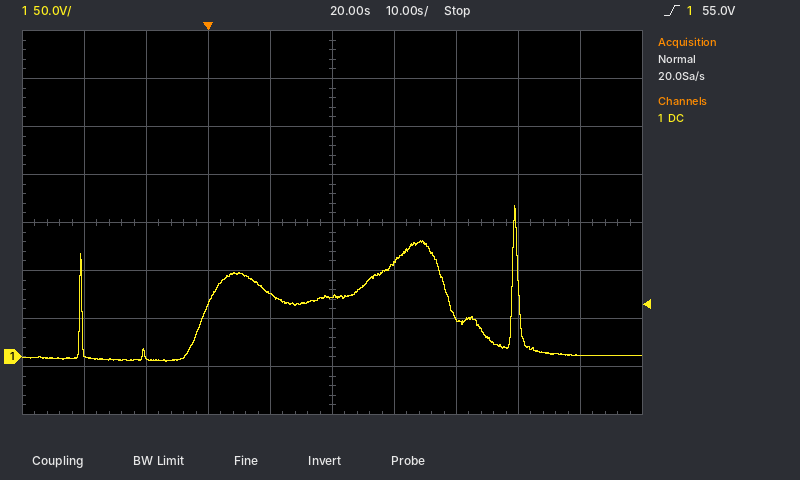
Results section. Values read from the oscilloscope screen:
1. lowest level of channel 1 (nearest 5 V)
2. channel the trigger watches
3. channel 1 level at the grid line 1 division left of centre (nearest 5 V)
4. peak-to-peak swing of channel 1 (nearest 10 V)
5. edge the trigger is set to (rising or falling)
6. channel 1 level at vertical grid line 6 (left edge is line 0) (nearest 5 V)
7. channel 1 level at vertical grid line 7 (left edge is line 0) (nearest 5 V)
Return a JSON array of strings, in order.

["-5 V", "channel 1", "65 V", "160 V", "rising", "100 V", "40 V"]
